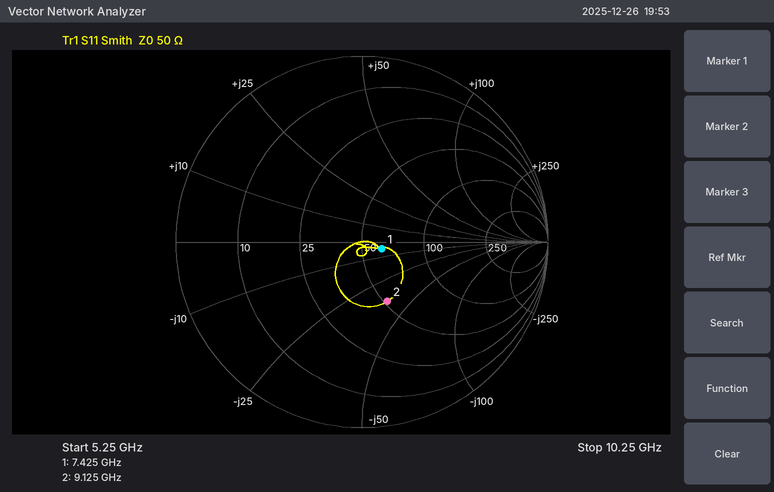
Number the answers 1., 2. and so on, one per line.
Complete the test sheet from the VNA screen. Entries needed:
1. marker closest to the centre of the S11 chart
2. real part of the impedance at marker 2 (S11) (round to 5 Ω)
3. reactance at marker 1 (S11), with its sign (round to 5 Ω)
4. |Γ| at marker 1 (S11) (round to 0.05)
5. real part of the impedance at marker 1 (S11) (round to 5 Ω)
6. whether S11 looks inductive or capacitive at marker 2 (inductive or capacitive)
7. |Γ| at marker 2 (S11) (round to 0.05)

1. marker 1
2. 50 Ω
3. -5 Ω
4. 0.10
5. 60 Ω
6. capacitive
7. 0.35
